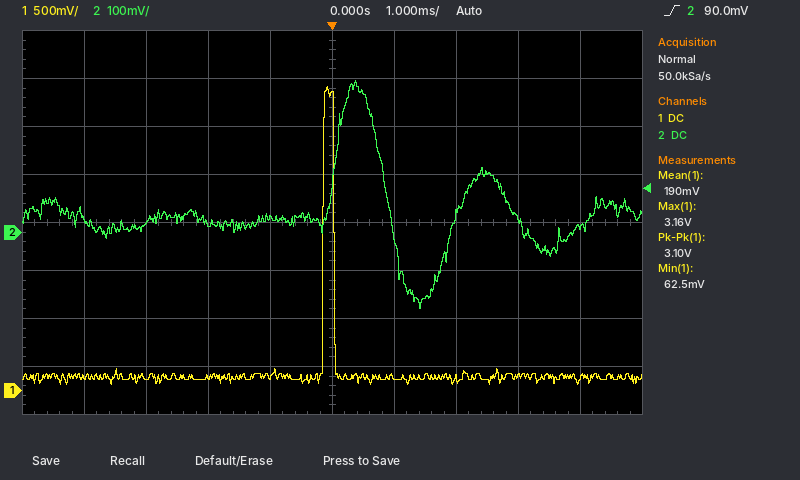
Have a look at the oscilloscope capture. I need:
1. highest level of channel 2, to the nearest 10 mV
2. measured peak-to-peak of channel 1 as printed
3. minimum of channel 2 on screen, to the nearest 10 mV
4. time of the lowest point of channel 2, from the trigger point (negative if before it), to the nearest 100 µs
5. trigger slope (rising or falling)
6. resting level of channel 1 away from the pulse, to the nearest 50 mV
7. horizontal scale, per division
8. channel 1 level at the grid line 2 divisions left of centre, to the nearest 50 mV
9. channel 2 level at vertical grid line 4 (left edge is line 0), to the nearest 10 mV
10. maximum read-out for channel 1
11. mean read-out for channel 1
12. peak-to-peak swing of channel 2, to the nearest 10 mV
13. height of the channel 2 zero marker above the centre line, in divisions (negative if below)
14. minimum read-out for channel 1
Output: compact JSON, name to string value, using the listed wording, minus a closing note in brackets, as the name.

{"highest level of channel 2, to the nearest 10 mV": "320 mV", "measured peak-to-peak of channel 1 as printed": "3.10 V", "minimum of channel 2 on screen, to the nearest 10 mV": "-160 mV", "time of the lowest point of channel 2, from the trigger point (negative if before it), to the nearest 100 µs": "+1.4 ms", "trigger slope": "rising", "resting level of channel 1 away from the pulse, to the nearest 50 mV": "150 mV", "horizontal scale, per division": "1 ms", "channel 1 level at the grid line 2 divisions left of centre, to the nearest 50 mV": "150 mV", "channel 2 level at vertical grid line 4 (left edge is line 0), to the nearest 10 mV": "30 mV", "maximum read-out for channel 1": "3.16 V", "mean read-out for channel 1": "190 mV", "peak-to-peak swing of channel 2, to the nearest 10 mV": "480 mV", "height of the channel 2 zero marker above the centre line, in divisions": "-0.2 div", "minimum read-out for channel 1": "62.5 mV"}
